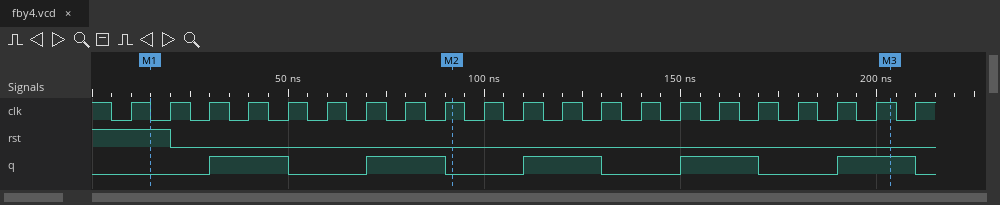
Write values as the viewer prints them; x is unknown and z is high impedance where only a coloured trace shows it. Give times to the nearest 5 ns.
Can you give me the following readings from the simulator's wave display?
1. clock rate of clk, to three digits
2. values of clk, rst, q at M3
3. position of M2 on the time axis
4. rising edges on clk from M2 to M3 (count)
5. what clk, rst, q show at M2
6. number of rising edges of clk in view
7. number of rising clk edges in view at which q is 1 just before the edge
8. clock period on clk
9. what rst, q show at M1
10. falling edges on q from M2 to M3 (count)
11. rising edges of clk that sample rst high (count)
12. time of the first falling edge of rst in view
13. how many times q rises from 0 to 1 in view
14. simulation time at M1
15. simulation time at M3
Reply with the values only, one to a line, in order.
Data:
100 MHz
clk=1, rst=0, q=1
90 ns
11
clk=1, rst=0, q=0
21
10
10 ns
rst=1, q=0
2
2
20 ns
5
15 ns
205 ns
